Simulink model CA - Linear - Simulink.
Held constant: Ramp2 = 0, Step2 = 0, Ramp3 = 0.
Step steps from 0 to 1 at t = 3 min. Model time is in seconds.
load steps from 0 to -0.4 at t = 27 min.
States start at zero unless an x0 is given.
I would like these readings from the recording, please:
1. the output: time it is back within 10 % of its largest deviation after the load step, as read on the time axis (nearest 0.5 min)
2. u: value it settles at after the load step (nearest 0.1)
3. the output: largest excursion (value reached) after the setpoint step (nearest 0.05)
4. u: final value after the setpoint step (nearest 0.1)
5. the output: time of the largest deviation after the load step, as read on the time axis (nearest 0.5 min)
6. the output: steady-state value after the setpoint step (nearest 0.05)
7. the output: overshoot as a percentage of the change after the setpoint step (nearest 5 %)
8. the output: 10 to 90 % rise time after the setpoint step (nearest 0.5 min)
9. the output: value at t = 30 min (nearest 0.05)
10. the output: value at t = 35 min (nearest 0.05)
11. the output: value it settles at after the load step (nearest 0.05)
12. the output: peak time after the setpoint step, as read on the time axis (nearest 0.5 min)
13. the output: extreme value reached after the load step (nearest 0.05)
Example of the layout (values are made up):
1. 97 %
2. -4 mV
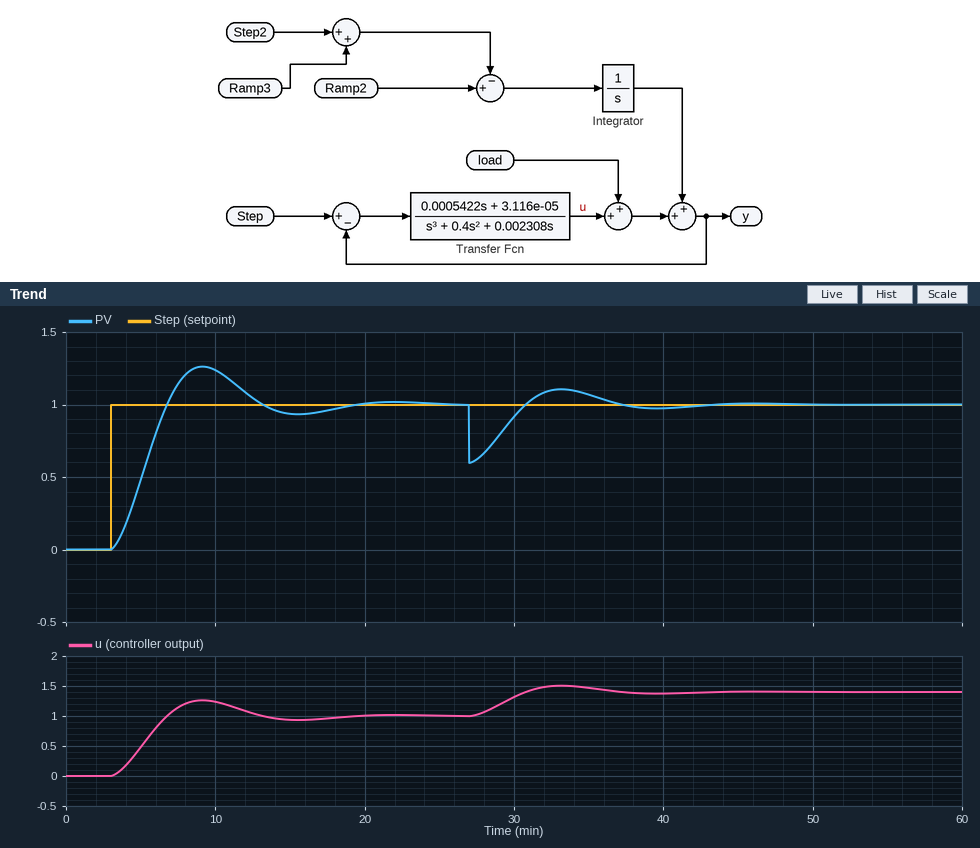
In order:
1. 36.0 min
2. 1.4
3. 1.25
4. 1.0
5. 27.0 min
6. 1.00
7. 25 %
8. 2.5 min
9. 0.90
10. 1.05
11. 1.00
12. 9.0 min
13. 0.60
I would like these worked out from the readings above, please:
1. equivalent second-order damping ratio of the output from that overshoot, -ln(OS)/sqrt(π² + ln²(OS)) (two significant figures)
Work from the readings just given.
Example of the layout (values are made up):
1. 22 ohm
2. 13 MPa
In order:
1. 0.40
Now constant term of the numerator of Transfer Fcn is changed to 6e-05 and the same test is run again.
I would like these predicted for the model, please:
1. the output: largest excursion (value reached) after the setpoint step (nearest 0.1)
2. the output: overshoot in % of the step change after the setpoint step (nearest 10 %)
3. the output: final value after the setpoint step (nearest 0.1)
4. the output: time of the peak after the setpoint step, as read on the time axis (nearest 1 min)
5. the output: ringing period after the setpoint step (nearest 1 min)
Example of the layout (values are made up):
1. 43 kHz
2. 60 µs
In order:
1. 1.4
2. 40 %
3. 1.0
4. 7 min
5. 9 min
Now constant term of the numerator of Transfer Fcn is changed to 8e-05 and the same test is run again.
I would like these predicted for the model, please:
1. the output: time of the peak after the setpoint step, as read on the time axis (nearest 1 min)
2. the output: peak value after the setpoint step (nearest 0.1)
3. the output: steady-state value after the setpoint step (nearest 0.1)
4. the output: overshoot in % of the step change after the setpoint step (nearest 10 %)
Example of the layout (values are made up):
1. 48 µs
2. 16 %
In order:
1. 7 min
2. 1.5
3. 1.0
4. 50 %
